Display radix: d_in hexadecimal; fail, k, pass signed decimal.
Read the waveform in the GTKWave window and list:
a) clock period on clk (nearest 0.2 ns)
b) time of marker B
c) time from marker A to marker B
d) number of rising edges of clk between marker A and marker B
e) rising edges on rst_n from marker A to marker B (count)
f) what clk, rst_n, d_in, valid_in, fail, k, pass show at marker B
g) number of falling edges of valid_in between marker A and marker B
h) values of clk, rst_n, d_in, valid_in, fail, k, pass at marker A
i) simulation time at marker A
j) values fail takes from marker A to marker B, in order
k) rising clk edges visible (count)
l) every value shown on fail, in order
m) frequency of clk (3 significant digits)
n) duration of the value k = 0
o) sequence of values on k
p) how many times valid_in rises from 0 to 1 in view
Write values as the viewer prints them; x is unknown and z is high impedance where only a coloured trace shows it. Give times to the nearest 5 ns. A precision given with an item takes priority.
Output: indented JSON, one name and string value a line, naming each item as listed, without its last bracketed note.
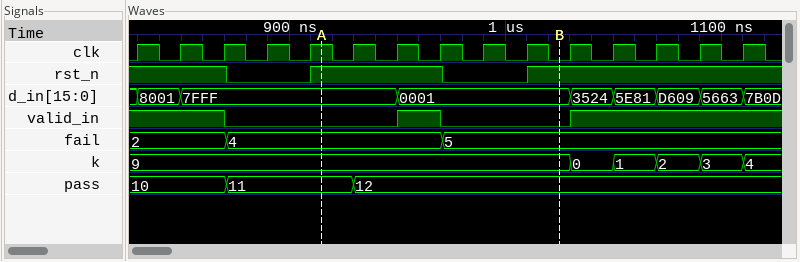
{
  "clock period on clk": "20 ns",
  "time of marker B": "1025 ns",
  "time from marker A to marker B": "110 ns",
  "number of rising edges of clk between marker A and marker B": "5",
  "rising edges on rst_n from marker A to marker B": "1",
  "what clk, rst_n, d_in, valid_in, fail, k, pass show at marker B": "clk=0, rst_n=1, d_in=0001, valid_in=0, fail=5, k=9, pass=12",
  "number of falling edges of valid_in between marker A and marker B": "1",
  "values of clk, rst_n, d_in, valid_in, fail, k, pass at marker A": "clk=1, rst_n=1, d_in=7FFF, valid_in=0, fail=4, k=9, pass=11",
  "simulation time at marker A": "915 ns",
  "values fail takes from marker A to marker B, in order": "4, 5",
  "rising clk edges visible": "15",
  "every value shown on fail, in order": "2, 4, 5",
  "frequency of clk": "50.0 MHz",
  "duration of the value k = 0": "20 ns",
  "sequence of values on k": "9, 0, 1, 2, 3, 4",
  "how many times valid_in rises from 0 to 1 in view": "2"
}
